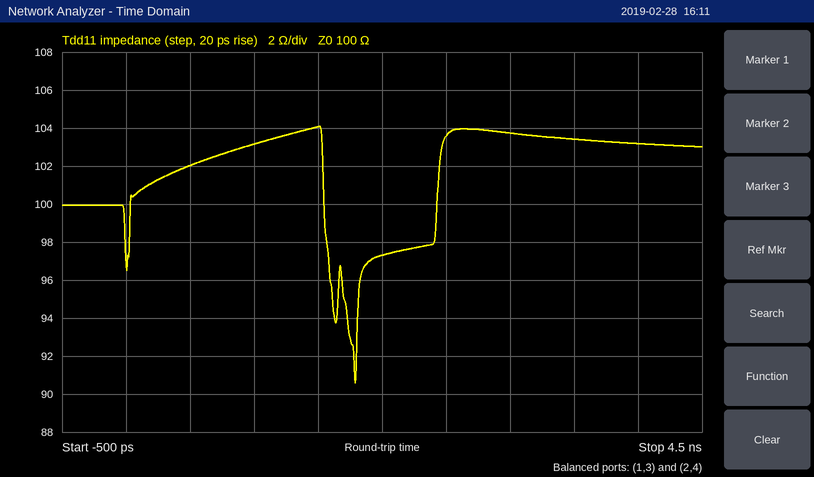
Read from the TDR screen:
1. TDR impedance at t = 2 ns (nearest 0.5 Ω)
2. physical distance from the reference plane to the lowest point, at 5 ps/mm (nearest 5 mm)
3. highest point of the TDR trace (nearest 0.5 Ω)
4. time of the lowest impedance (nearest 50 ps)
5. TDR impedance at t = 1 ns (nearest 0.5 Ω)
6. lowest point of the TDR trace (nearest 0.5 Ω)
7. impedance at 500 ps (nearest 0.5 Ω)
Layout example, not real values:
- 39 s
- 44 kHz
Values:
- 97.5 Ω
- 180 mm
- 104.0 Ω
- 1.80 ns
- 103.0 Ω
- 90.5 Ω
- 102.0 Ω
